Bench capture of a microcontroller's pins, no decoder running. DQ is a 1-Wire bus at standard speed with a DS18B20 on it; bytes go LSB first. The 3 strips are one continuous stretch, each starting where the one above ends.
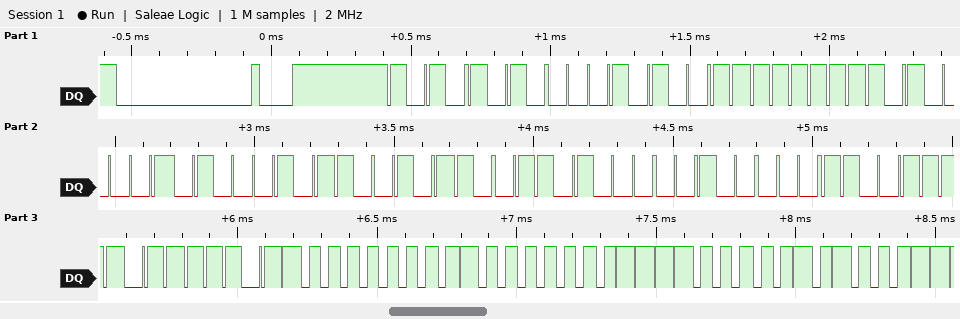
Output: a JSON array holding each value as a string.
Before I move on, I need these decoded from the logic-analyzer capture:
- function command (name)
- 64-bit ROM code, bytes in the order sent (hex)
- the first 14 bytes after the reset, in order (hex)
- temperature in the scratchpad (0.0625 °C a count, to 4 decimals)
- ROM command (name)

["Read Scratchpad", "28 FF 85 A2 69 16 04 F3", "55 28 FF 85 A2 69 16 04 F3 BE 01 02 1E 14", "32.0625 °C", "Match ROM"]
